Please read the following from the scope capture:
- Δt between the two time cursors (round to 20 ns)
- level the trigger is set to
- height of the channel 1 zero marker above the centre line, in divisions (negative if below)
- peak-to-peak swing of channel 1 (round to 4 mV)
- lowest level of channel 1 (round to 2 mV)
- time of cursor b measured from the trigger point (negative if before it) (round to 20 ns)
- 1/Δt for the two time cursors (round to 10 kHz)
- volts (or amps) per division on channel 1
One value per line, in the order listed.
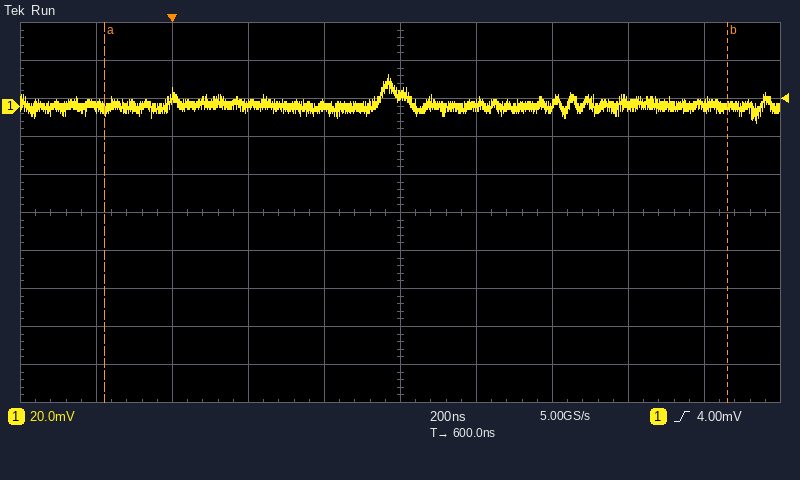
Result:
1.64 µs
4.00 mV
+2.8 div
24 mV
-8 mV
+1.46 µs
610 kHz
20 mV
